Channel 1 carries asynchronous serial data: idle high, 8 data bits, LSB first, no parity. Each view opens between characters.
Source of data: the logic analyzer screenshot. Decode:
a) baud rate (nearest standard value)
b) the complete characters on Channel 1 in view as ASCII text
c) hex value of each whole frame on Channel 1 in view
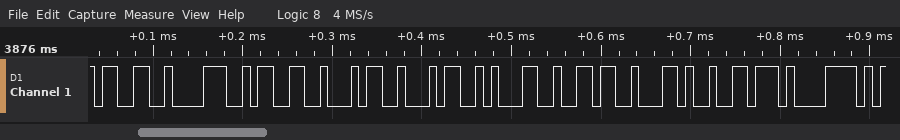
115200 baud
"3834416,vx"
33, 38, 33, 34, 34, 31, 36, 2C, 76, 78
